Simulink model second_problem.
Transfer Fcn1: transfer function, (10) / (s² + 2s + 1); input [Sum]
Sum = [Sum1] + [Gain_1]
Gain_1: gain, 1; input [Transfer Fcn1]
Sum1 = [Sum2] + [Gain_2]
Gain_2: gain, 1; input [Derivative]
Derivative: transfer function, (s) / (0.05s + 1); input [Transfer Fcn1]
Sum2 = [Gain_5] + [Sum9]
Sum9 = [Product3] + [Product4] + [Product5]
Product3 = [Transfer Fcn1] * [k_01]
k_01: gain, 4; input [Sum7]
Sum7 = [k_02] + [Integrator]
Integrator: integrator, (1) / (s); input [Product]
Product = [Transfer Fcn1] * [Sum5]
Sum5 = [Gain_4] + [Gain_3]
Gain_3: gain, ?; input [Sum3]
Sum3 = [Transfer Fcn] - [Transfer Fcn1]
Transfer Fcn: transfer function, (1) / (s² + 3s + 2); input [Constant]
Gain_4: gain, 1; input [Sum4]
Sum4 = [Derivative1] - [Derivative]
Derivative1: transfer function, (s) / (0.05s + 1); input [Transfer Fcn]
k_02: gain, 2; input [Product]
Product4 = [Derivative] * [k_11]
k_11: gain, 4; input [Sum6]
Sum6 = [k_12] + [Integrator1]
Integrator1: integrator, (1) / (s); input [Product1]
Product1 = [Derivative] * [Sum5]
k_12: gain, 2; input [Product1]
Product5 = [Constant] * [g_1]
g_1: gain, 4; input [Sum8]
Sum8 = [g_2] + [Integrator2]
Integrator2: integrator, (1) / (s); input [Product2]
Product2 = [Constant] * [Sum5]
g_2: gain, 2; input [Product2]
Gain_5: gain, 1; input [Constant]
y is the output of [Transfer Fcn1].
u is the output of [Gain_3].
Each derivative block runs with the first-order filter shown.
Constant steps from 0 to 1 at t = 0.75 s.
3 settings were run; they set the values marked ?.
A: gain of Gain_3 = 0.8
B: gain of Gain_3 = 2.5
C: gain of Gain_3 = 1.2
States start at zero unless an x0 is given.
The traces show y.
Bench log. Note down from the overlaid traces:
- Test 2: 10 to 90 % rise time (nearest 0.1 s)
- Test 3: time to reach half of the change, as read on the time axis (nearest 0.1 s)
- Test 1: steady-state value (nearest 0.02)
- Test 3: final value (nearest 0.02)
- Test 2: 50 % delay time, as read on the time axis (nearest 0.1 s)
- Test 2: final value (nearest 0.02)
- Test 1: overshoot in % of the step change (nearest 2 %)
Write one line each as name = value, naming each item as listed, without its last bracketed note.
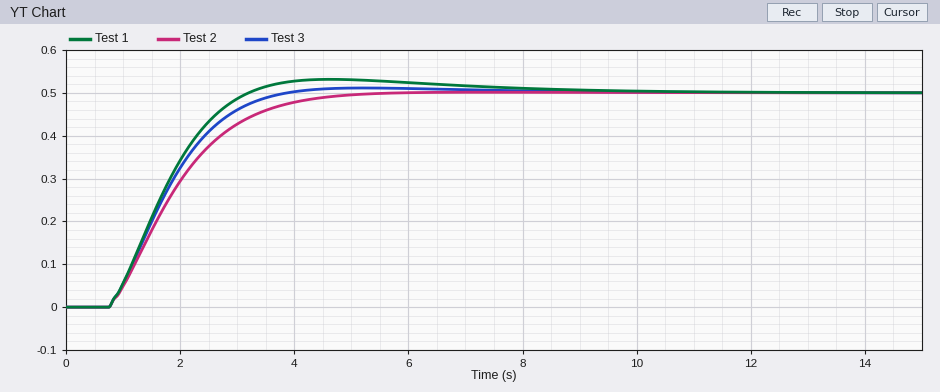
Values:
Test 2: 10 to 90 % rise time = 2.3 s
Test 3: time to reach half of the change, as read on the time axis = 1.7 s
Test 1: steady-state value = 0.50
Test 3: final value = 0.50
Test 2: 50 % delay time, as read on the time axis = 1.8 s
Test 2: final value = 0.50
Test 1: overshoot in % of the step change = 6 %
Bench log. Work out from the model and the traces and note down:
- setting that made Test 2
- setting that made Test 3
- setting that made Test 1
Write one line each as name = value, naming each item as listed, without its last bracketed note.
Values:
setting that made Test 2 = B
setting that made Test 3 = C
setting that made Test 1 = A
